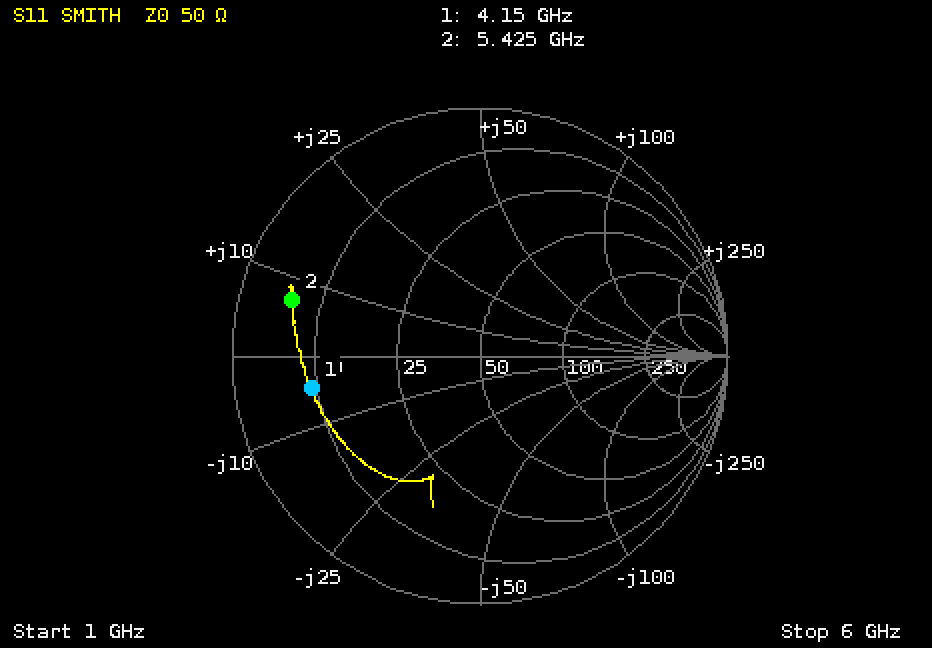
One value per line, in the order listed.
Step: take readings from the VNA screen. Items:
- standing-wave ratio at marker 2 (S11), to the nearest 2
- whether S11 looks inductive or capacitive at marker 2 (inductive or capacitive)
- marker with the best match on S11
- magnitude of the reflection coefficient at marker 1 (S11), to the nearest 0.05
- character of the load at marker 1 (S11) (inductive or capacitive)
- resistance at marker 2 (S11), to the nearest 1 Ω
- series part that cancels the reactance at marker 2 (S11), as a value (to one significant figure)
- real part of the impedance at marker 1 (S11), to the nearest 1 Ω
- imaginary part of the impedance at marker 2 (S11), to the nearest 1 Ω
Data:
8
inductive
marker 1
0.70
capacitive
6 Ω
4 pF
9 Ω
+7 Ω
